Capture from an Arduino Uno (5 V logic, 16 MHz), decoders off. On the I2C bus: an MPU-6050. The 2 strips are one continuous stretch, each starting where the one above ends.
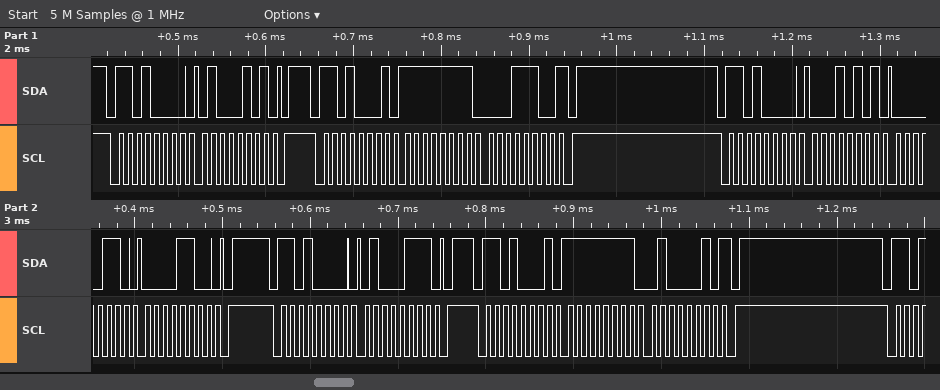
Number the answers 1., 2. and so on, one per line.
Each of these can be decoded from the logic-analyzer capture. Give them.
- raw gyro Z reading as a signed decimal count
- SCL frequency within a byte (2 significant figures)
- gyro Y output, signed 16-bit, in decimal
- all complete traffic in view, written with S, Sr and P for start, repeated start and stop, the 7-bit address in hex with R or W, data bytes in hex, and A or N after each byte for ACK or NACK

1. -190
2. 100 kHz
3. -228
4. S 68W A 45 A P S 68R A FF A 1C N P S 68W A 15 A 06 A 0C A P S 68W A 47 A P S 68R A FF A 42 N P
